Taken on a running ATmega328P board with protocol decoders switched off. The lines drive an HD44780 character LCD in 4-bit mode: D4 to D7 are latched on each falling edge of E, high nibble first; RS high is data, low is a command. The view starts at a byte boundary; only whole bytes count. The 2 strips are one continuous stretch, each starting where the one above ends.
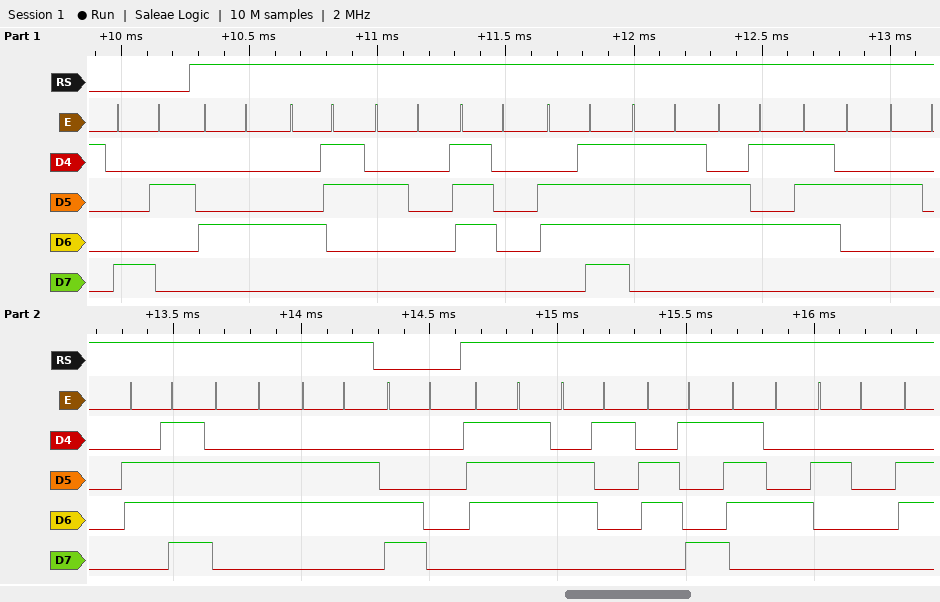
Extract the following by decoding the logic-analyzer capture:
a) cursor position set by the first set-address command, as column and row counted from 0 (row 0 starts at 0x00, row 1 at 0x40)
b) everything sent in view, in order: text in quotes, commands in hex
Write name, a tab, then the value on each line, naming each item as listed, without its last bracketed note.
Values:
cursor position set by the first set-address command, as column and row counted from 0	column 2, row 0
everything sent in view, in order: text in quotes, commands in hex	0x82 "DC power off" 0xC0 "wait "
